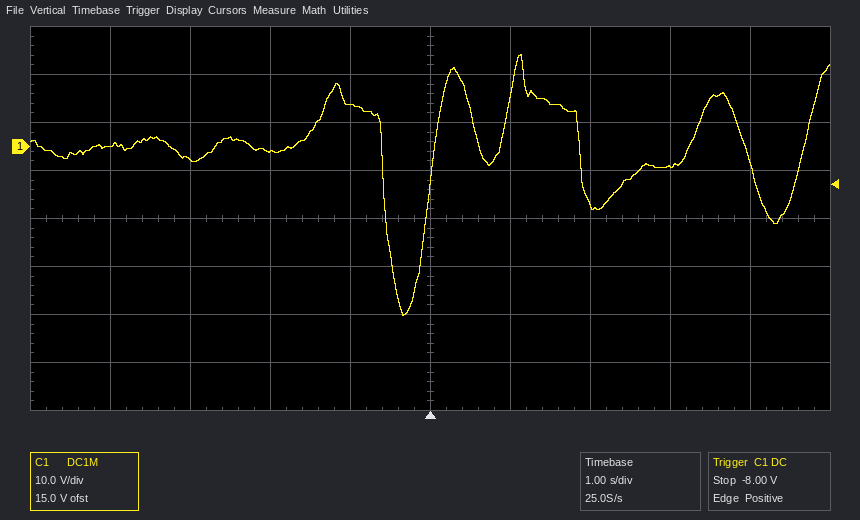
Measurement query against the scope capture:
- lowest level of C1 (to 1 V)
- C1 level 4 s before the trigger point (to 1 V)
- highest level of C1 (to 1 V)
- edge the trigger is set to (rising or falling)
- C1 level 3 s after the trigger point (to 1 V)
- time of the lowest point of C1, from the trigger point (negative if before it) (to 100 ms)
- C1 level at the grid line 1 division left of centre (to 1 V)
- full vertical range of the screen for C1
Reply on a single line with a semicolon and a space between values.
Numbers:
-35 V; 0 V; 19 V; rising; -4 V; -300 ms; 9 V; 80 V
